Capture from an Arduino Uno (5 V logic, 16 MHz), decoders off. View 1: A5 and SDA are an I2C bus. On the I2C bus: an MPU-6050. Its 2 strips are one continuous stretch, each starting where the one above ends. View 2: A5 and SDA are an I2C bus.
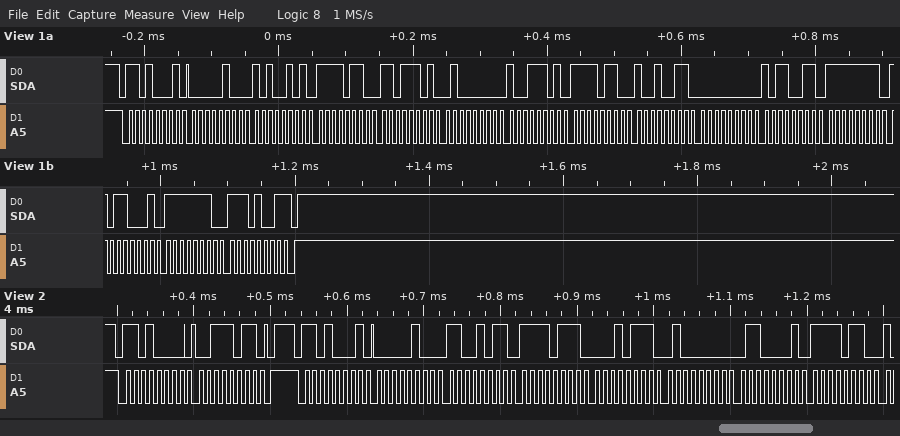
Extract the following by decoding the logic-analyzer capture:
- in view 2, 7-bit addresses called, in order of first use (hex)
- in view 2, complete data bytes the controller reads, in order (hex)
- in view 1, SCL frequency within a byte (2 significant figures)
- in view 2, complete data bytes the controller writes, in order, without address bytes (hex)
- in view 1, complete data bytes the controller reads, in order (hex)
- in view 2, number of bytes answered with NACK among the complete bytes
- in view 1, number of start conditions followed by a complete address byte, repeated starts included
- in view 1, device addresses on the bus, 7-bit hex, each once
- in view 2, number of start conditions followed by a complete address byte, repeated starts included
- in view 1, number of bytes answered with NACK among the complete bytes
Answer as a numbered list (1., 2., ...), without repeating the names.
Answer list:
1. 0x68
2. 04 CB F7 17 40 61 F6
3. 100 kHz
4. 3B
5. 04 A5 F6 DD 40 9D F6 93 00 B3 FF B1 FE E9
6. 0
7. 1
8. 0x68
9. 2
10. 1
